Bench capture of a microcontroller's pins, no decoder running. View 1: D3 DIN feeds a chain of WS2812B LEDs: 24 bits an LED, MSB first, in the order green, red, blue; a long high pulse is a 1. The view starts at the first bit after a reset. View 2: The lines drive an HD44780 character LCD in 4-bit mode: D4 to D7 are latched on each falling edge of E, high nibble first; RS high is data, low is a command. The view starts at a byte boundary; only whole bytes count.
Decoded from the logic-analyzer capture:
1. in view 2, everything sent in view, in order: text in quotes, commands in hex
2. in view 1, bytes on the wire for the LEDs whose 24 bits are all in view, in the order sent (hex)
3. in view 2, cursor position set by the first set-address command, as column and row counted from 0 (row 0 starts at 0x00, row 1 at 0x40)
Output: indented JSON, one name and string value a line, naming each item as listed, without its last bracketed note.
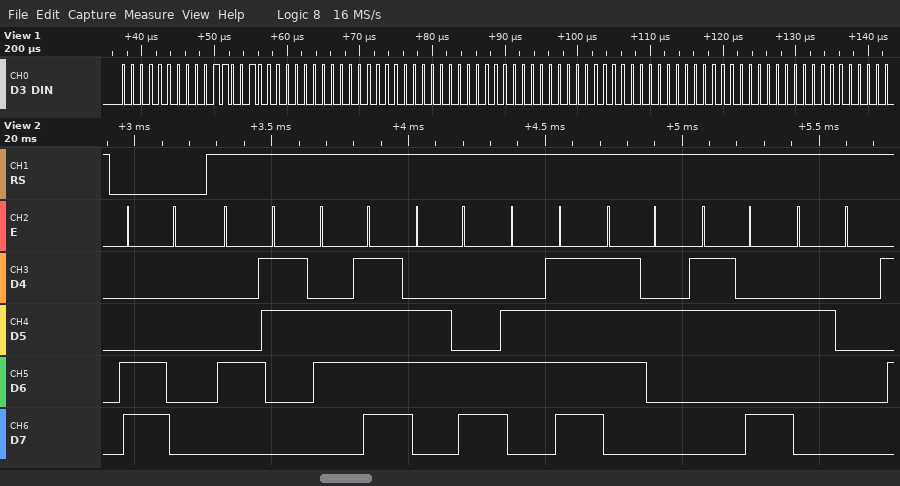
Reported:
{
  "in view 2, everything sent in view, in order: text in quotes, commands in hex": "0xC0 \"Color: \"",
  "in view 1, bytes on the wire for the LEDs whose 24 bits are all in view, in the order sent": "00 32 00 00 00 00 00 00 00",
  "in view 2, cursor position set by the first set-address command, as column and row counted from 0": "column 0, row 1"
}
